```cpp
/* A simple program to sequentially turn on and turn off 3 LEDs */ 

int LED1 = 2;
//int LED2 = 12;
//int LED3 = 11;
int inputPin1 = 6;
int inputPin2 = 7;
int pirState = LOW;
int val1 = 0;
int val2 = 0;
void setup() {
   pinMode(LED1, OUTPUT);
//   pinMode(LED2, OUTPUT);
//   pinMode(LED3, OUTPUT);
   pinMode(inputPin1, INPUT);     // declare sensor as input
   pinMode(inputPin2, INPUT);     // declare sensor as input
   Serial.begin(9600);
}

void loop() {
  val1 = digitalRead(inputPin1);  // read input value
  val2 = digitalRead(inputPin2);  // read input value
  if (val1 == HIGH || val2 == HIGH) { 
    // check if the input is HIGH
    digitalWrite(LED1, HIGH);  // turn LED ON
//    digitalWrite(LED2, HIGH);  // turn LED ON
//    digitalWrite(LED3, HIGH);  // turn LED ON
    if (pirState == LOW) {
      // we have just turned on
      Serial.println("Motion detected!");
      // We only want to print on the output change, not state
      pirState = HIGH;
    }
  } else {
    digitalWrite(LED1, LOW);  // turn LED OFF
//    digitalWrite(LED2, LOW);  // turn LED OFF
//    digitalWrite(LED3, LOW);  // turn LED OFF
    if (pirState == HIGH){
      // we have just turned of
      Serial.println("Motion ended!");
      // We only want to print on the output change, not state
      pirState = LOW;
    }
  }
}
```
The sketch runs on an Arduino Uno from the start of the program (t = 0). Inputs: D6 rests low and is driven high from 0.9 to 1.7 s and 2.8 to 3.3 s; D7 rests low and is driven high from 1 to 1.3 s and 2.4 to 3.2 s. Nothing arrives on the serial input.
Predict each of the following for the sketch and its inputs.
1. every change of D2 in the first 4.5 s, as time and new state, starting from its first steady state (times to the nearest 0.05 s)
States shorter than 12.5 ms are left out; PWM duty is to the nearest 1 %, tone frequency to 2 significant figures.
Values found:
0 s low; 0.9 s high; 1.7 s low; 2.4 s high; 3.3 s low
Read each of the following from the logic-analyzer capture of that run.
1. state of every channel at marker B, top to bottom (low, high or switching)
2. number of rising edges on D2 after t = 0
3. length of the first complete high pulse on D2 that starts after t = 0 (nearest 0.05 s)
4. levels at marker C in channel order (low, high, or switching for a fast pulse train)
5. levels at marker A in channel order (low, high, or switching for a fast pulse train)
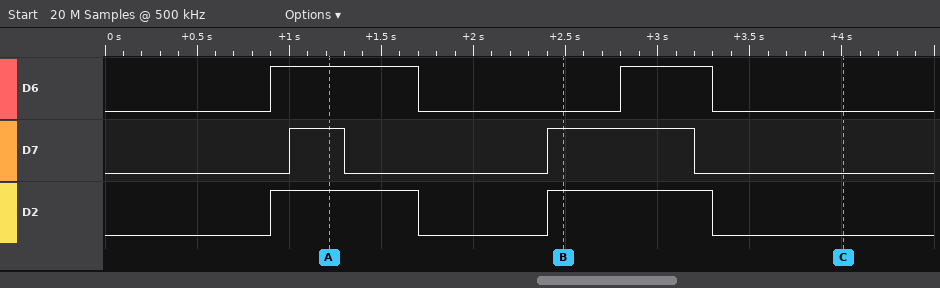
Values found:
D6 low, D7 high, D2 high
2
0.80 s
D6 low, D7 low, D2 low
D6 high, D7 high, D2 high
